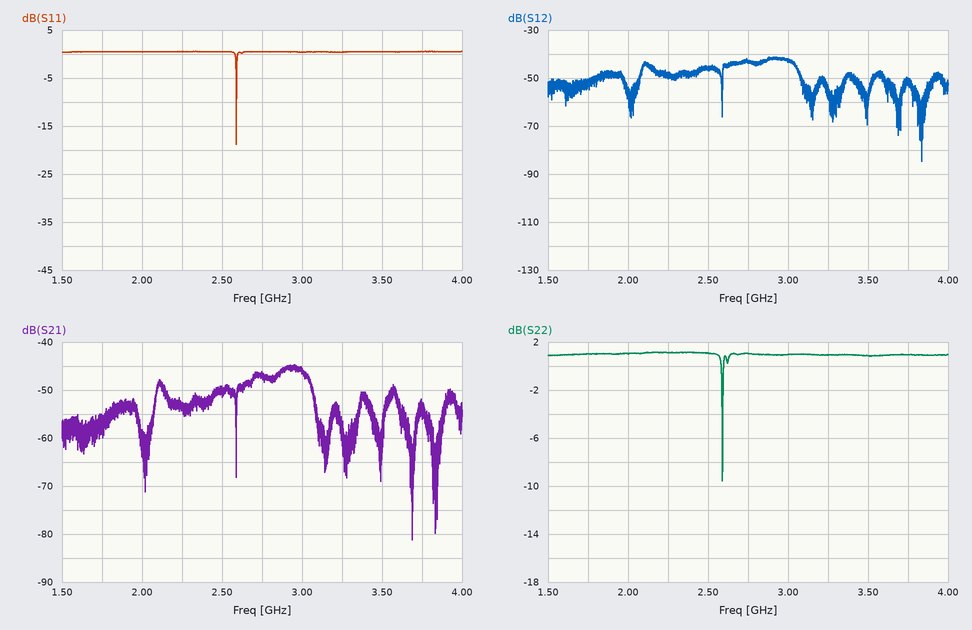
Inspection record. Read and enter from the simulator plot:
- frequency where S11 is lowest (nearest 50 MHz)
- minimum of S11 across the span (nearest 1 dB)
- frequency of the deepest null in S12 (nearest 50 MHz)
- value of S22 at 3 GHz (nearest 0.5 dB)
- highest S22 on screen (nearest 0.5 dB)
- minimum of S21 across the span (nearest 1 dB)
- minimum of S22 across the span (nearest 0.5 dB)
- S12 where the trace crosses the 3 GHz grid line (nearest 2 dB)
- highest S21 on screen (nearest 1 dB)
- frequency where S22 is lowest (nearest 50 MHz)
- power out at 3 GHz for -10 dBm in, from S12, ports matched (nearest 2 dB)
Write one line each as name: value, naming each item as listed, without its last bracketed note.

frequency where S11 is lowest: 2.60 GHz
minimum of S11 across the span: -19 dB
frequency of the deepest null in S12: 3.85 GHz
value of S22 at 3 GHz: 1.0 dB
highest S22 on screen: 1.0 dB
minimum of S21 across the span: -81 dB
minimum of S22 across the span: -9.5 dB
S12 where the trace crosses the 3 GHz grid line: -42 dB
highest S21 on screen: -45 dB
frequency where S22 is lowest: 2.60 GHz
power out at 3 GHz for -10 dBm in, from S12, ports matched: -52 dBm
